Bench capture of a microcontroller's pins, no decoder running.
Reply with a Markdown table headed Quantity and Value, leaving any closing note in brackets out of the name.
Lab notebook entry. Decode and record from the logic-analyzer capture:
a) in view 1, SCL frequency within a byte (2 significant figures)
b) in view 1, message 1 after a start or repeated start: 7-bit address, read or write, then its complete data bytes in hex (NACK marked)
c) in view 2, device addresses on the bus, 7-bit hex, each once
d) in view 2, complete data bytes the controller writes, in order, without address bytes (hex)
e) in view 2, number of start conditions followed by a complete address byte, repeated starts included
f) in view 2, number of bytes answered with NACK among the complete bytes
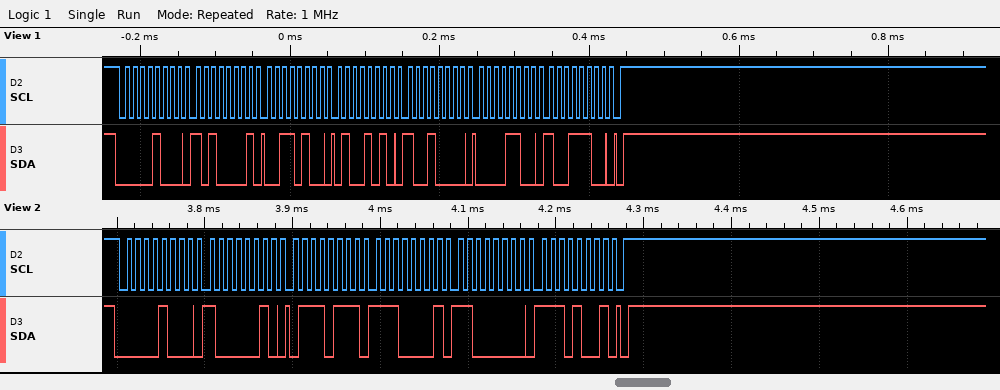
| Quantity | Value |
|---|---|
| in view 1, SCL frequency within a byte | 100 kHz |
| in view 1, message 1 after a start or repeated start: 7-bit address, read or write, then its complete data bytes in hex | 0x04 write: A1 34 4A 90 0C 9C |
| in view 2, device addresses on the bus, 7-bit hex, each once | 0x04 |
| in view 2, complete data bytes the controller writes, in order, without address bytes | 82 77 E1 C0 E9 |
| in view 2, number of start conditions followed by a complete address byte, repeated starts included | 1 |
| in view 2, number of bytes answered with NACK among the complete bytes | 0 |
